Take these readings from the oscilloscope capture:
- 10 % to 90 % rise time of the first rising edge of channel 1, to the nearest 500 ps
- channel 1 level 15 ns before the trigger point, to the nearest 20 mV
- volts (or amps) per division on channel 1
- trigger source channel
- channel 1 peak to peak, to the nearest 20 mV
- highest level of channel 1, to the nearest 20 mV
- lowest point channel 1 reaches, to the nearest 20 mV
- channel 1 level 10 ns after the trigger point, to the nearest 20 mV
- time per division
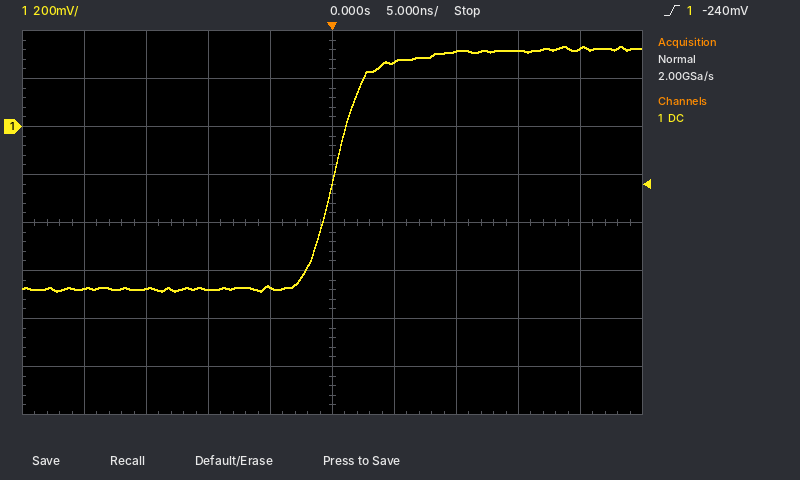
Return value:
4.5 ns
-680 mV
200 mV
channel 1
1.02 V
340 mV
-680 mV
320 mV
5 ns
